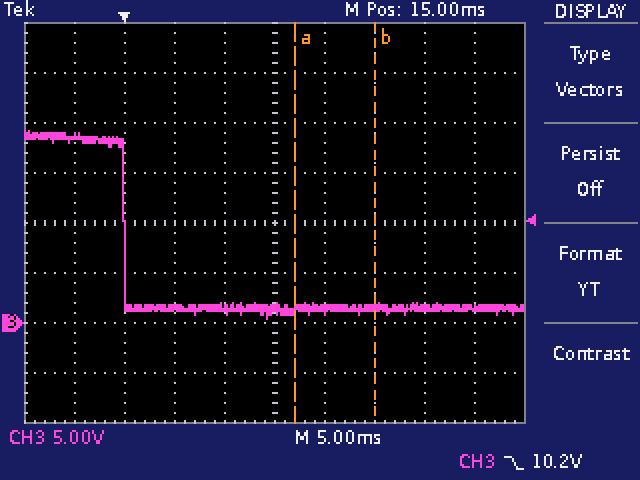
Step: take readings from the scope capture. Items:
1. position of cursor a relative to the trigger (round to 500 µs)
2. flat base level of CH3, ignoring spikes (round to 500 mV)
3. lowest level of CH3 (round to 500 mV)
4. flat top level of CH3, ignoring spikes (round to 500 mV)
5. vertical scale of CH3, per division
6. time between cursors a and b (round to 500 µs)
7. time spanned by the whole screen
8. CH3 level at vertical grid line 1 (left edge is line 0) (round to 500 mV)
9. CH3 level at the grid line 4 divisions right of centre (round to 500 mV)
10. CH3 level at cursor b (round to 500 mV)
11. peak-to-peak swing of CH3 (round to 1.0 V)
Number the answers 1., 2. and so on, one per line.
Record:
1. +17.0 ms
2. 1.5 V
3. 500 mV
4. 18.5 V
5. 5 V
6. 8.0 ms
7. 50 ms
8. 18.5 V
9. 1.5 V
10. 1.5 V
11. 19.0 V
